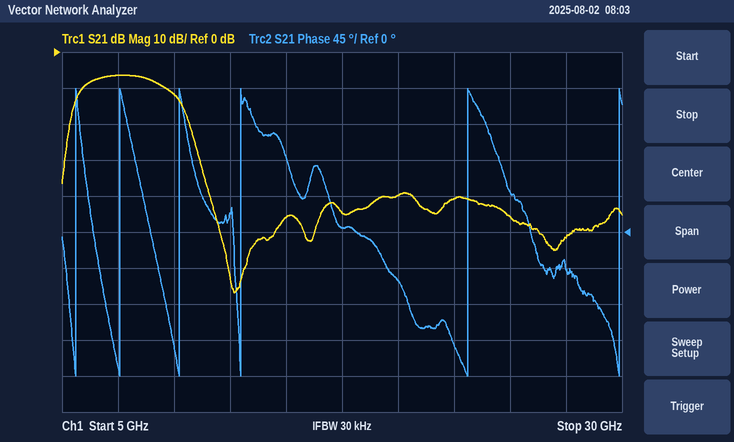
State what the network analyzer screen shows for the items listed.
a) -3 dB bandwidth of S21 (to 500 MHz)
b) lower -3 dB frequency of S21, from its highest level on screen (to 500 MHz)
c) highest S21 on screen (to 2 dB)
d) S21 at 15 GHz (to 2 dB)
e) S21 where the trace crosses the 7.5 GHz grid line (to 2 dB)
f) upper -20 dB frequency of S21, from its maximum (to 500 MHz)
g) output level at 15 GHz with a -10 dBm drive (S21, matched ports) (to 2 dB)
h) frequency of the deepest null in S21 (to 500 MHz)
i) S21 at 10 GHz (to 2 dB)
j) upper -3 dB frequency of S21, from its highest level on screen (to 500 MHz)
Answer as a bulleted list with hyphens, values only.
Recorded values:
- 3.5 GHz
- 6.0 GHz
- -6 dB
- -46 dB
- -6 dB
- 11.0 GHz
- -56 dBm
- 12.5 GHz
- -12 dB
- 9.5 GHz
